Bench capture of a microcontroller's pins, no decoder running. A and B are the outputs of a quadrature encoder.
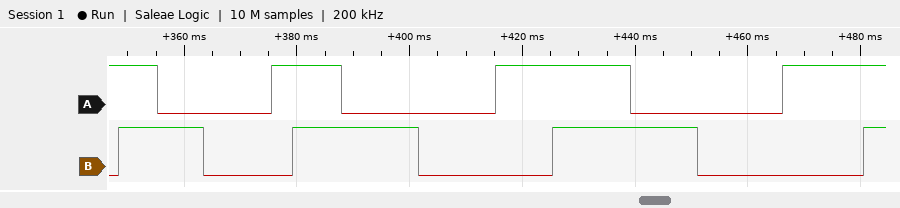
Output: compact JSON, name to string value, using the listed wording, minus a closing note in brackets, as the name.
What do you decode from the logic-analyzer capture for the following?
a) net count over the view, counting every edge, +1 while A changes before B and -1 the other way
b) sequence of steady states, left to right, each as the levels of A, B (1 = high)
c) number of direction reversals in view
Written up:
{"net count over the view, counting every edge, +1 while A changes before B and -1 the other way": "+13", "sequence of steady states, left to right, each as the levels of A, B": "10 11 01 00 10 11 01 00 10 11 01 00 10 11", "number of direction reversals in view": "0"}
